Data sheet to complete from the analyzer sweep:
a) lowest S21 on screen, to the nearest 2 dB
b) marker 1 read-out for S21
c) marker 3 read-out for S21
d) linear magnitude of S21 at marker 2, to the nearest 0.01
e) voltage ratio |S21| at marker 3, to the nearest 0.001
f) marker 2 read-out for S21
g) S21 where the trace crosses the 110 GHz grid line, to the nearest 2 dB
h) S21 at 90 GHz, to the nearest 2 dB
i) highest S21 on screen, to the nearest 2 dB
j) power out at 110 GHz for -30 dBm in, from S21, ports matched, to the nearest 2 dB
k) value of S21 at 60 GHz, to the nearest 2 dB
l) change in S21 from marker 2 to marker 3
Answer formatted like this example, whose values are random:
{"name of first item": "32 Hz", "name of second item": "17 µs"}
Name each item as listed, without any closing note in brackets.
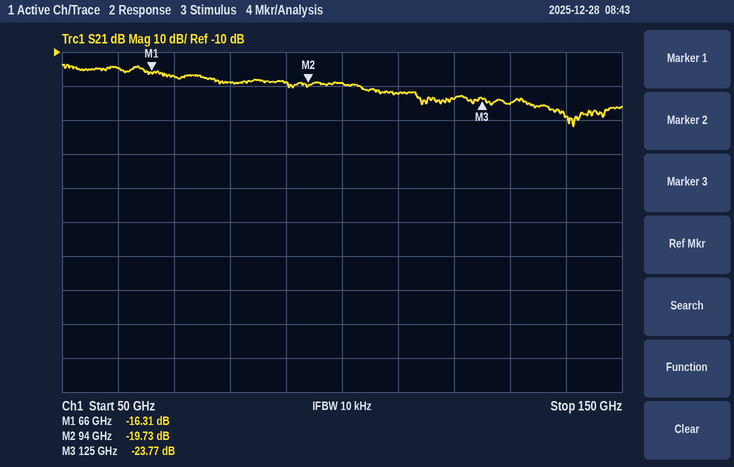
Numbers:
{"lowest S21 on screen, to the nearest 2 dB": "-32 dB", "marker 1 read-out for S21": "-16.31 dB", "marker 3 read-out for S21": "-23.77 dB", "linear magnitude of S21 at marker 2, to the nearest 0.01": "0.10", "voltage ratio |S21| at marker 3, to the nearest 0.001": "0.065", "marker 2 read-out for S21": "-19.73 dB", "S21 where the trace crosses the 110 GHz grid line, to the nearest 2 dB": "-22 dB", "S21 at 90 GHz, to the nearest 2 dB": "-18 dB", "highest S21 on screen, to the nearest 2 dB": "-14 dB", "power out at 110 GHz for -30 dBm in, from S21, ports matched, to the nearest 2 dB": "-52 dBm", "value of S21 at 60 GHz, to the nearest 2 dB": "-14 dB", "change in S21 from marker 2 to marker 3": "-4.04 dB"}
